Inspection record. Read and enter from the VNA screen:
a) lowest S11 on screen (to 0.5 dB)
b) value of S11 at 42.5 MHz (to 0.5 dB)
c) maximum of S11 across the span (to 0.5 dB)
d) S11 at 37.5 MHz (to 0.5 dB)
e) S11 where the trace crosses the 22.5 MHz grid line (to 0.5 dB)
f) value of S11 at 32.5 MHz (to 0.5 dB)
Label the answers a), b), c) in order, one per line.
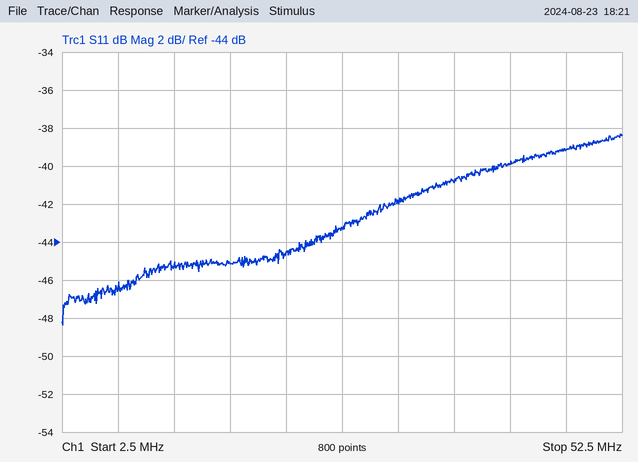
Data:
a) -48.5 dB
b) -40.0 dB
c) -38.5 dB
d) -41.0 dB
e) -44.5 dB
f) -42.0 dB
